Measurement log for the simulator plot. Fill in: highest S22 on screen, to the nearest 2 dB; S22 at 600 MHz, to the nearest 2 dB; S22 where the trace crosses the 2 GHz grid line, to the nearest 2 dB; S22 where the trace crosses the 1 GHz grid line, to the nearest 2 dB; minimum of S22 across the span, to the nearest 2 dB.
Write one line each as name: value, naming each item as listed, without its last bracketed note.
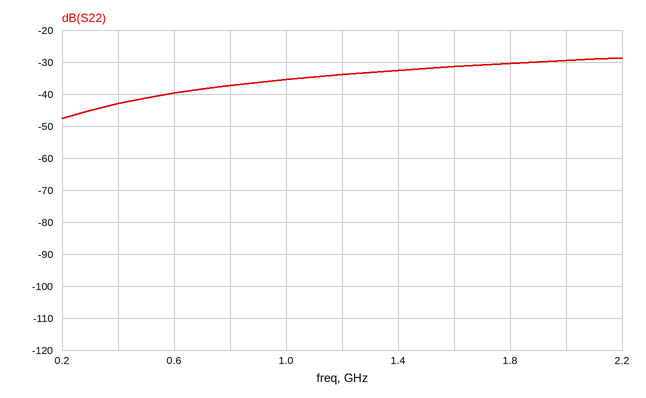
highest S22 on screen, to the nearest 2 dB: -28 dB
S22 at 600 MHz, to the nearest 2 dB: -40 dB
S22 where the trace crosses the 2 GHz grid line, to the nearest 2 dB: -30 dB
S22 where the trace crosses the 1 GHz grid line, to the nearest 2 dB: -36 dB
minimum of S22 across the span, to the nearest 2 dB: -48 dB
